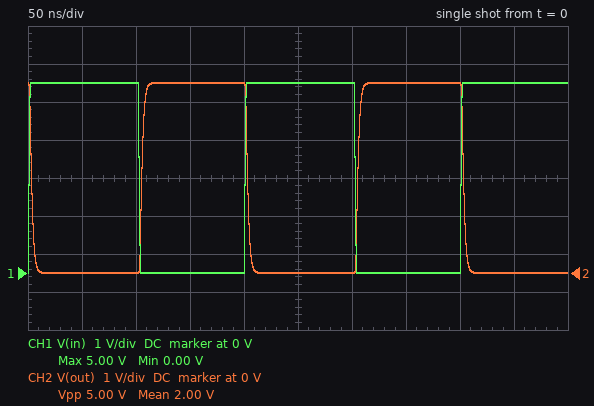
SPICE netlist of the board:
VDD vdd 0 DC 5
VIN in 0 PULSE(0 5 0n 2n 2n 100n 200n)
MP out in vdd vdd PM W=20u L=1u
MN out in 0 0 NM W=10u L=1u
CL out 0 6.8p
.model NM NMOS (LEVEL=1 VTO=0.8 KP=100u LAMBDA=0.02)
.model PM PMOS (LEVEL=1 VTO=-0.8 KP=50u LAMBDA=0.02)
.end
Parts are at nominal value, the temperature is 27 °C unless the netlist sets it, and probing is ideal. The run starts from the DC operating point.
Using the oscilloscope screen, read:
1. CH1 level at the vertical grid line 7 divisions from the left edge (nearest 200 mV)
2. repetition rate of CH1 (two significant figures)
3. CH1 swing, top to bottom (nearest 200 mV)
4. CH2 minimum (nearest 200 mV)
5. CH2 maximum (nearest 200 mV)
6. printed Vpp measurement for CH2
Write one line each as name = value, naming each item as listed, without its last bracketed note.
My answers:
CH1 level at the vertical grid line 7 divisions from the left edge = 0 V
repetition rate of CH1 = 5.0 MHz
CH1 swing, top to bottom = 5.0 V
CH2 minimum = 0 V
CH2 maximum = 5.0 V
printed Vpp measurement for CH2 = 5.00 V
